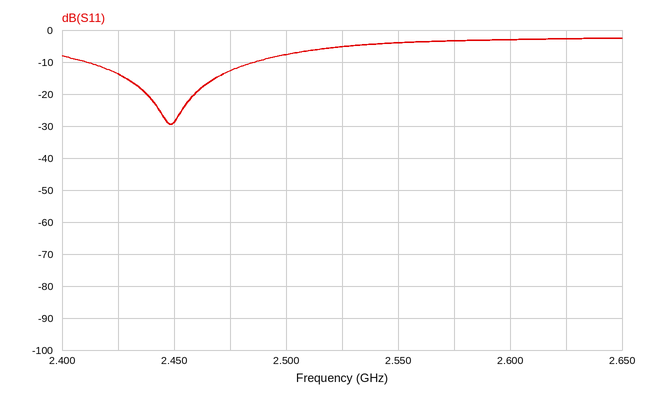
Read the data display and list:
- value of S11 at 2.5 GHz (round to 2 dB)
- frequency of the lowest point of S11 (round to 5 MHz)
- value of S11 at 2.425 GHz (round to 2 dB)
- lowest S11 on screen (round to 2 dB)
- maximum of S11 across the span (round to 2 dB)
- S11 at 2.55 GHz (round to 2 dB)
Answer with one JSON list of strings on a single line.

["-8 dB", "2.450 GHz", "-14 dB", "-30 dB", "-2 dB", "-4 dB"]
